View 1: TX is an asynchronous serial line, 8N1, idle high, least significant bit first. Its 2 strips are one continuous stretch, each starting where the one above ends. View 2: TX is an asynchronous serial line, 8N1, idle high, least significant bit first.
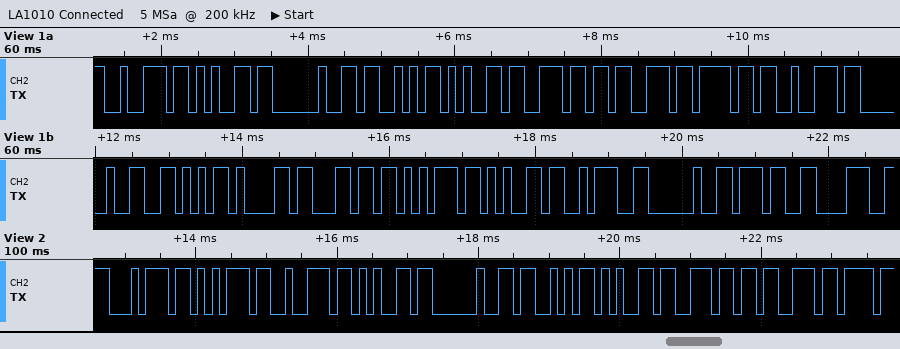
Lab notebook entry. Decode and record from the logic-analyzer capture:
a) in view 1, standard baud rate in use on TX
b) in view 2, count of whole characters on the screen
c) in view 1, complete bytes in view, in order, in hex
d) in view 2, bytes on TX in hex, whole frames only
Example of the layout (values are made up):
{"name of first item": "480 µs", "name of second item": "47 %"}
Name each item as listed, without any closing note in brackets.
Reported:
{"in view 1, standard baud rate in use on TX": "9600 baud", "in view 2, count of whole characters on the screen": "9", "in view 1, complete bytes in view, in order, in hex": "72 65 20 53 65 6E 73 6F 72 20 56 61 6C 75 65 3A 20 37 38", "in view 2, bytes on TX in hex, whole frames only": "74 75 72 65 20 53 65 6E 73"}
